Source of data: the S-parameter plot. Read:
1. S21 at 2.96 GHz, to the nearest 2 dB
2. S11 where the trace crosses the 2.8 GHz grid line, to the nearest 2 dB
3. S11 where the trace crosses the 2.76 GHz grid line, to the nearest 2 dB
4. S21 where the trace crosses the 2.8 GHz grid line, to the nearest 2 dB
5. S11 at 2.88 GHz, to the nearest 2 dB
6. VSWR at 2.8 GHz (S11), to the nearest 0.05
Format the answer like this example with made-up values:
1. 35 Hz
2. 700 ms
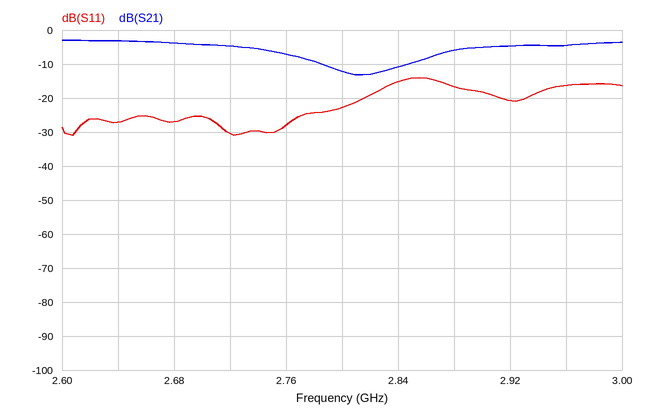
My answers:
1. -4 dB
2. -22 dB
3. -28 dB
4. -12 dB
5. -16 dB
6. 1.15
